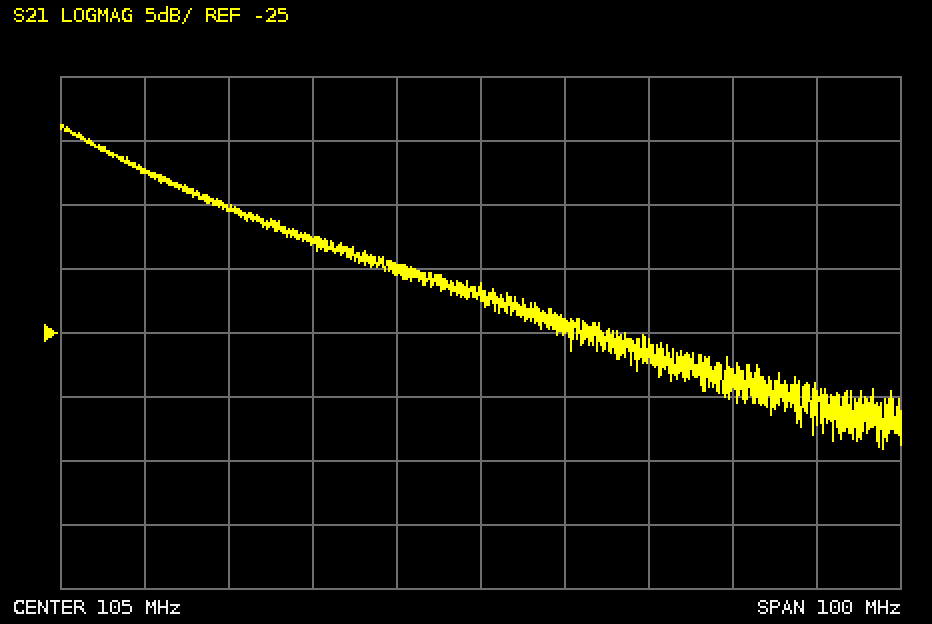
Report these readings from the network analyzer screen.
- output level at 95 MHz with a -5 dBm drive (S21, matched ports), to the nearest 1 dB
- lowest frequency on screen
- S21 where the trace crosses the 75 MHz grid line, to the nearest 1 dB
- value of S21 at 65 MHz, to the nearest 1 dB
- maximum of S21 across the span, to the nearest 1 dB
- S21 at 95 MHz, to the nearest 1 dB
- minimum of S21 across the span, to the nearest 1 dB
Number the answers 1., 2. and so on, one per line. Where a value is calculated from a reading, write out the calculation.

1. -5 dBm + (-20 dB) = -25 dBm
2. 55 MHz
3. -15 dB
4. -12 dB
5. -9 dB
6. -20 dB
7. -34 dB
